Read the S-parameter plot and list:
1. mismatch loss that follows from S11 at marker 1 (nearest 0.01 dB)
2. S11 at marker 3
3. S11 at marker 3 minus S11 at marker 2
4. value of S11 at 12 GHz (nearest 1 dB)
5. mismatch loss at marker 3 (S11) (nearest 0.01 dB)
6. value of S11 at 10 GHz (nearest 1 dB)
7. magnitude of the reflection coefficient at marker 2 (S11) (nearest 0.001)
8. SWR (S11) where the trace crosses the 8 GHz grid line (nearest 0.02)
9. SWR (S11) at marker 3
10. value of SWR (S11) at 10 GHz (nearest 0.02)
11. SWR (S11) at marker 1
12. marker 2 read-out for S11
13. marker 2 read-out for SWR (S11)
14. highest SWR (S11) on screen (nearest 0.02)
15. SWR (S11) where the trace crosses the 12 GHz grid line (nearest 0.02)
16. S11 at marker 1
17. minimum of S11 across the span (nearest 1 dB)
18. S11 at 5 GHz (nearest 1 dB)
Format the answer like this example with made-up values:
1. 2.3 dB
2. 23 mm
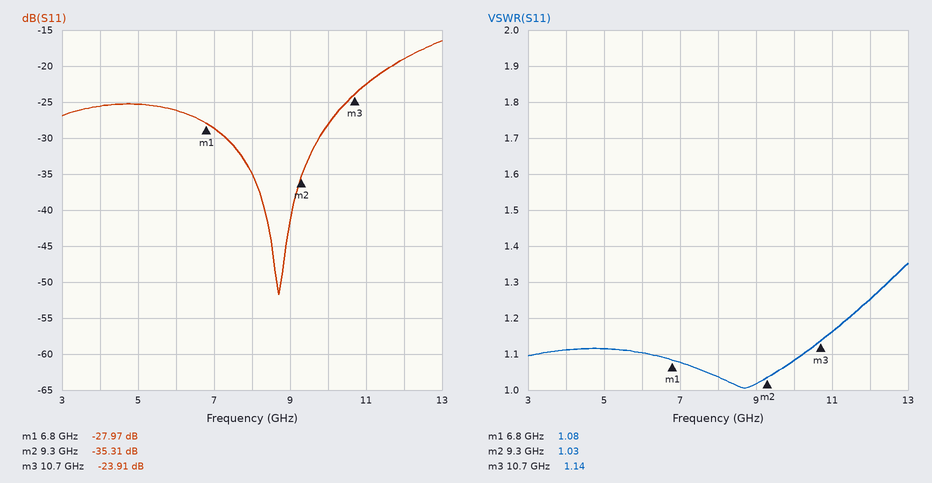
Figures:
1. 0.01 dB
2. -23.91 dB
3. 11.40 dB
4. -19 dB
5. 0.02 dB
6. -28 dB
7. 0.017
8. 1.04
9. 1.14
10. 1.08
11. 1.08
12. -35.31 dB
13. 1.03
14. 1.36
15. 1.26
16. -27.97 dB
17. -52 dB
18. -25 dB
